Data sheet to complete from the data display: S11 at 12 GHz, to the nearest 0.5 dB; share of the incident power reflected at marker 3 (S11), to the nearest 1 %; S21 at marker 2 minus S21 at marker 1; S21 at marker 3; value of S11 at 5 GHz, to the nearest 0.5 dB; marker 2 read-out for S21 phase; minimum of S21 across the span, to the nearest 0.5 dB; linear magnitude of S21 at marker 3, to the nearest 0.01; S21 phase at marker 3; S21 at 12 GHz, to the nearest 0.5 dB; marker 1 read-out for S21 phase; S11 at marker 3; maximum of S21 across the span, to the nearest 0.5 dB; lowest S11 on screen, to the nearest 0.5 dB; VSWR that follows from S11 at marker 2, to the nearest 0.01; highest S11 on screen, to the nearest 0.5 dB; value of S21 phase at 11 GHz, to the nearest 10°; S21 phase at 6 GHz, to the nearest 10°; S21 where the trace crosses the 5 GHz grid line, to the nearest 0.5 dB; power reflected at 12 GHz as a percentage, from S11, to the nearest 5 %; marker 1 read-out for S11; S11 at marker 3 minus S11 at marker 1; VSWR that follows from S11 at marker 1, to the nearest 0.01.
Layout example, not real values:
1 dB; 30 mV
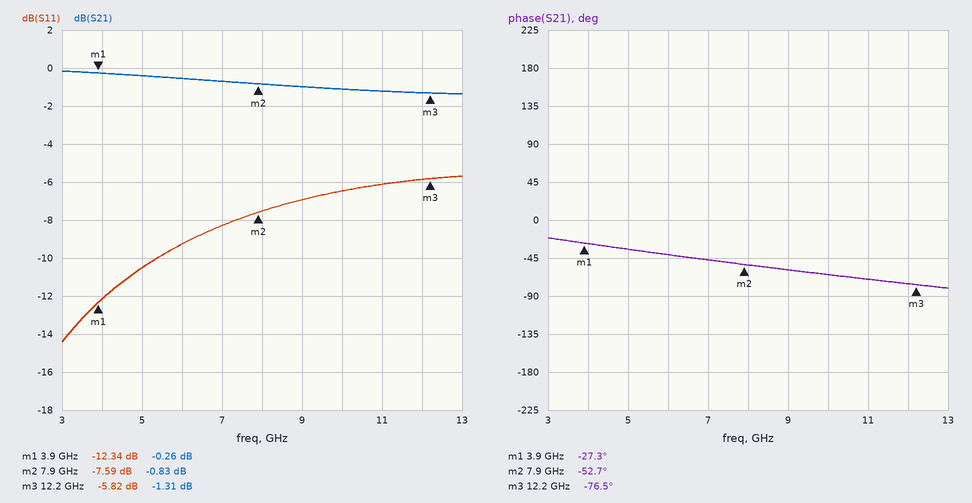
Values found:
-6.0 dB; 26 %; -0.57 dB; -1.31 dB; -10.5 dB; -52.7°; -1.5 dB; 0.86; -76.5°; -1.5 dB; -27.3°; -5.82 dB; 0.0 dB; -14.5 dB; 2.43; -5.5 dB; -70°; -40°; -0.5 dB; 25 %; -12.34 dB; 6.52 dB; 1.64
